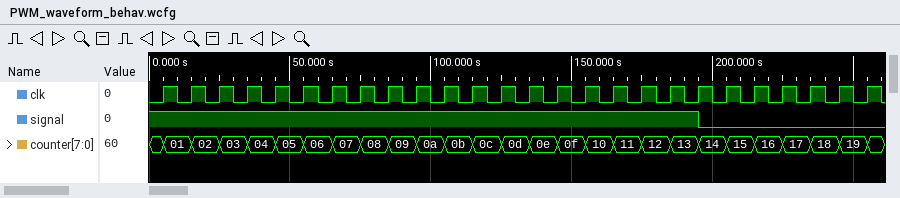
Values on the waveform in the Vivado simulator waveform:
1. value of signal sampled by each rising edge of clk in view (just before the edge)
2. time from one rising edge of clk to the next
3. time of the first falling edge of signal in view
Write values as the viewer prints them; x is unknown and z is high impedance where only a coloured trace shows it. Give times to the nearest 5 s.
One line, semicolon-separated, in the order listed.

1 1 1 1 1 1 1 1 1 1 1 1 1 1 1 1 1 1 1 1 0 0 0 0 0 0; 10 s; 195 s
